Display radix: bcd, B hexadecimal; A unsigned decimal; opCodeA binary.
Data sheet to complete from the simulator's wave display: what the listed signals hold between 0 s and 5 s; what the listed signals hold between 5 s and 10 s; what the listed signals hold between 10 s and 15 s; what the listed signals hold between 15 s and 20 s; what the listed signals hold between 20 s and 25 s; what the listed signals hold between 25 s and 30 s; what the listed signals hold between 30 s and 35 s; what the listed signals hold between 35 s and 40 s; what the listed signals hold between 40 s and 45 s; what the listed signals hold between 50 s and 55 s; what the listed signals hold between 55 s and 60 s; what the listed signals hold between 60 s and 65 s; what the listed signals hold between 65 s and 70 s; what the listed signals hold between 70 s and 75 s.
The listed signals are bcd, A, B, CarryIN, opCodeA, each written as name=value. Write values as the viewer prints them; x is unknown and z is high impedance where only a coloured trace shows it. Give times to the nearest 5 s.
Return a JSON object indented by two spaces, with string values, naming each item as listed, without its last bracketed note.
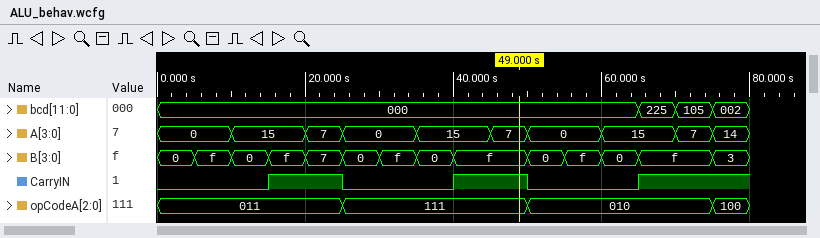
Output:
{
  "what the listed signals hold between 0 s and 5 s": "bcd=000, A=0, B=0, CarryIN=0, opCodeA=011",
  "what the listed signals hold between 5 s and 10 s": "bcd=000, A=0, B=f, CarryIN=0, opCodeA=011",
  "what the listed signals hold between 10 s and 15 s": "bcd=000, A=15, B=0, CarryIN=0, opCodeA=011",
  "what the listed signals hold between 15 s and 20 s": "bcd=000, A=15, B=f, CarryIN=1, opCodeA=011",
  "what the listed signals hold between 20 s and 25 s": "bcd=000, A=7, B=7, CarryIN=1, opCodeA=011",
  "what the listed signals hold between 25 s and 30 s": "bcd=000, A=0, B=0, CarryIN=0, opCodeA=111",
  "what the listed signals hold between 30 s and 35 s": "bcd=000, A=0, B=f, CarryIN=0, opCodeA=111",
  "what the listed signals hold between 35 s and 40 s": "bcd=000, A=15, B=0, CarryIN=0, opCodeA=111",
  "what the listed signals hold between 40 s and 45 s": "bcd=000, A=15, B=f, CarryIN=1, opCodeA=111",
  "what the listed signals hold between 50 s and 55 s": "bcd=000, A=0, B=0, CarryIN=0, opCodeA=010",
  "what the listed signals hold between 55 s and 60 s": "bcd=000, A=0, B=f, CarryIN=0, opCodeA=010",
  "what the listed signals hold between 60 s and 65 s": "bcd=000, A=15, B=0, CarryIN=0, opCodeA=010",
  "what the listed signals hold between 65 s and 70 s": "bcd=225, A=15, B=f, CarryIN=1, opCodeA=010",
  "what the listed signals hold between 70 s and 75 s": "bcd=105, A=7, B=f, CarryIN=1, opCodeA=010"
}
